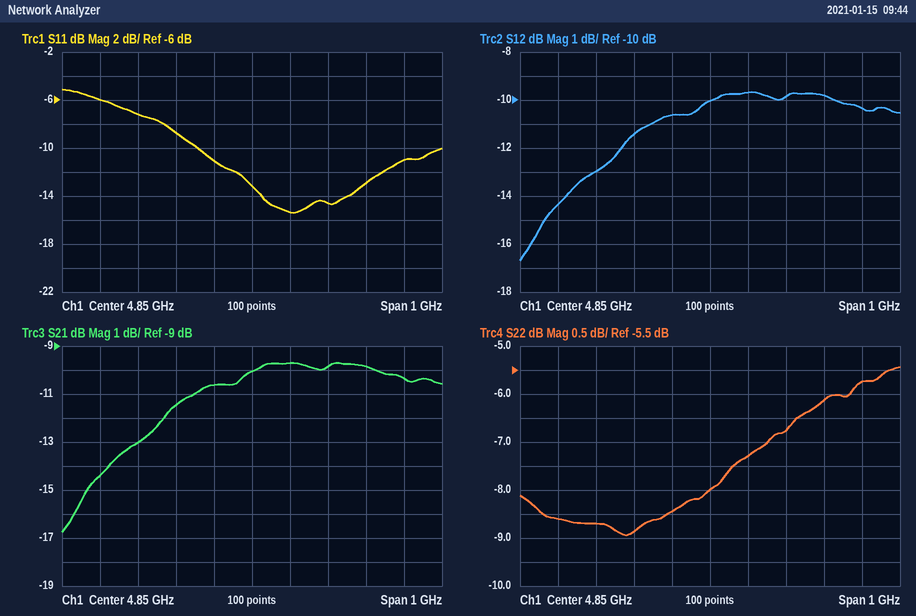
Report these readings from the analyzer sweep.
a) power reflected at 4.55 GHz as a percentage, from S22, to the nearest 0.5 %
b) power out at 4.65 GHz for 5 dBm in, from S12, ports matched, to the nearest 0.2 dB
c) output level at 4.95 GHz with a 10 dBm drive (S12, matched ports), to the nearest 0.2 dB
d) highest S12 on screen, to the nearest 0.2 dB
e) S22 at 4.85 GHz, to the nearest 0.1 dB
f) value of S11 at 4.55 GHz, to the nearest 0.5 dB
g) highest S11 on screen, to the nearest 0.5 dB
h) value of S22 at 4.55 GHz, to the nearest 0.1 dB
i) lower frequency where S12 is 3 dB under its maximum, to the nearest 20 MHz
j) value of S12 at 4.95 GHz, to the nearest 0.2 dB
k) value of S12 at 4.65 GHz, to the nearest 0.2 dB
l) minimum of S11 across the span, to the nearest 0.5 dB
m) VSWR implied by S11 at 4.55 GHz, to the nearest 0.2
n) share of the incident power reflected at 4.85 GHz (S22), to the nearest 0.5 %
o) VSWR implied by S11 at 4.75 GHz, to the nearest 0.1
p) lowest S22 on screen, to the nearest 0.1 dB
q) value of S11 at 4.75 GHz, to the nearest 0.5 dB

13.5 %
-6.4 dBm
0.4 dBm
-9.6 dB
-8.0 dB
-7.0 dB
-5.0 dB
-8.7 dB
4.58 GHz
-9.6 dB
-11.4 dB
-15.5 dB
2.6
16.0 %
1.8
-8.9 dB
-11.0 dB
